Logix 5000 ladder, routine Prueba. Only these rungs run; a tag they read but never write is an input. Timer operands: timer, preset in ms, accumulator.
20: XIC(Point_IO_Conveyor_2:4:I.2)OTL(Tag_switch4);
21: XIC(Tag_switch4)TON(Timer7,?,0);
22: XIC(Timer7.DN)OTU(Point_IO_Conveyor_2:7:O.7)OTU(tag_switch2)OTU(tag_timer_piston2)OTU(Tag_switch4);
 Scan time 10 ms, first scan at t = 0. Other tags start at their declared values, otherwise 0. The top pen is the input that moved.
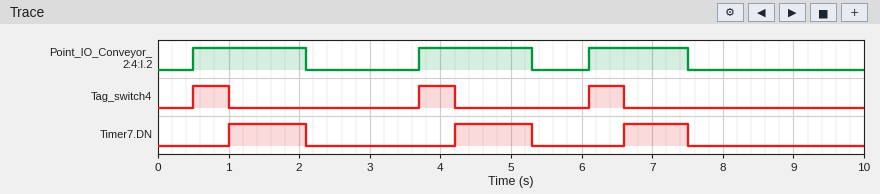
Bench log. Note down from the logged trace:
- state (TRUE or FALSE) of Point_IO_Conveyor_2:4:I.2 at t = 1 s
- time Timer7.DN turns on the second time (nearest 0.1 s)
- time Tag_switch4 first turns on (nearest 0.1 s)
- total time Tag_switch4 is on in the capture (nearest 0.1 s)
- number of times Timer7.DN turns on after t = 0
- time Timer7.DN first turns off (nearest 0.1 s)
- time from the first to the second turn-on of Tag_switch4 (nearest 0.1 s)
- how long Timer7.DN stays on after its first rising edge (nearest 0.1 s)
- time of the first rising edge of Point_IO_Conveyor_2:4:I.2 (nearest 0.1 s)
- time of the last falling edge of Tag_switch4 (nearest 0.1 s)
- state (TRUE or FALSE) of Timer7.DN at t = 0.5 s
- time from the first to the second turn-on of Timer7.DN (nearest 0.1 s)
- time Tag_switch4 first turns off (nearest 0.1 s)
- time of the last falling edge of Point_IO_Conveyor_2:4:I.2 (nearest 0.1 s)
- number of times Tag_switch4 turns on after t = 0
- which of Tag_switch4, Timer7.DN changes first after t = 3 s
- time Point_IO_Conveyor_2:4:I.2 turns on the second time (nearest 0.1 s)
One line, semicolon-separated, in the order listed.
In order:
TRUE; 4.2 s; 0.5 s; 1.5 s; 3; 2.1 s; 3.2 s; 1.1 s; 0.5 s; 6.6 s; FALSE; 3.2 s; 1.0 s; 7.5 s; 3; Tag_switch4; 3.7 s
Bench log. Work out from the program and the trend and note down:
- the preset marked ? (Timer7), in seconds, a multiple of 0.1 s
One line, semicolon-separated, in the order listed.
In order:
0.5 s
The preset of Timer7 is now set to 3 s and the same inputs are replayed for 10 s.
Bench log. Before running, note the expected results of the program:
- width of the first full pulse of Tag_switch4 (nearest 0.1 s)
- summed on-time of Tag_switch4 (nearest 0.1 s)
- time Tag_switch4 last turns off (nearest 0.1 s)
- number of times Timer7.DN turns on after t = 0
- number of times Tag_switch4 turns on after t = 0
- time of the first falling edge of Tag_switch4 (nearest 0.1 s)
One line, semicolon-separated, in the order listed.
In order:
3.0 s; 6.0 s; 6.7 s; 2; 2; 3.5 s
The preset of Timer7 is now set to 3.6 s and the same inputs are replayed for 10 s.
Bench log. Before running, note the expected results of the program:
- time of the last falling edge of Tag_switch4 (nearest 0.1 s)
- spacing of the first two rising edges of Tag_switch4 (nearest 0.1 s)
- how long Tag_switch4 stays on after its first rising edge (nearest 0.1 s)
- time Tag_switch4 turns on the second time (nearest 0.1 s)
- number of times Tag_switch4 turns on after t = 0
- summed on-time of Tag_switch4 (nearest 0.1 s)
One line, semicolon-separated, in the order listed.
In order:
9.7 s; 5.6 s; 3.6 s; 6.1 s; 2; 7.2 s
